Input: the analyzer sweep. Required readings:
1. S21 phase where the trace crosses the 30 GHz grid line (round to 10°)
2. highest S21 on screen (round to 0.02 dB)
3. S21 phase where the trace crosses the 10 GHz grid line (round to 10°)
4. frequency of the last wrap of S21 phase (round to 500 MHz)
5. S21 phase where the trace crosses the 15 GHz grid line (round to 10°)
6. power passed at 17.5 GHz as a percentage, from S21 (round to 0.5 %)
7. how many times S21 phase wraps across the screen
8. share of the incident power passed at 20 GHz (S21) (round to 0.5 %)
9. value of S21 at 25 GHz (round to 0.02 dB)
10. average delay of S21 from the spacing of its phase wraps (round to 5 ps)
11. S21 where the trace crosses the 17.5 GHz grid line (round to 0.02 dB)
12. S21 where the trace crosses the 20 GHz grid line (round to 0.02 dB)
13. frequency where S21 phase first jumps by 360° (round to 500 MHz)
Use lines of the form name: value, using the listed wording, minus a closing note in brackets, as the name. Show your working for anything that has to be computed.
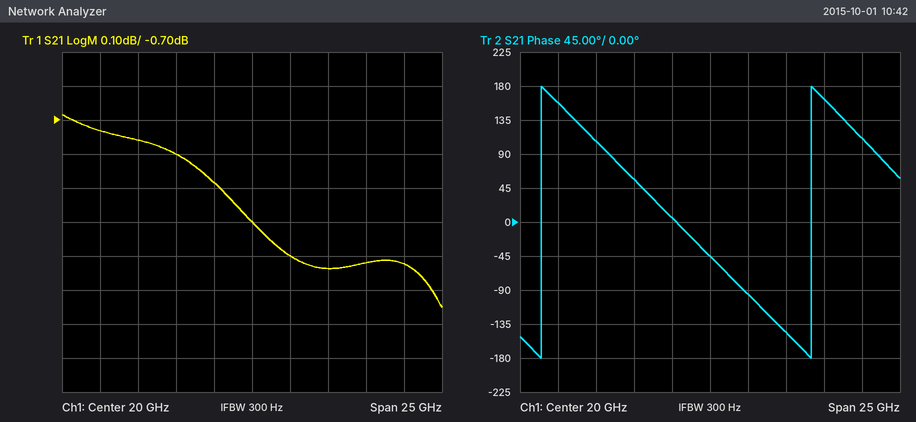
S21 phase where the trace crosses the 30 GHz grid line: 110°
highest S21 on screen: -0.68 dB
S21 phase where the trace crosses the 10 GHz grid line: 160°
frequency of the last wrap of S21 phase: 26.5 GHz
S21 phase where the trace crosses the 15 GHz grid line: 60°
power passed at 17.5 GHz as a percentage, from S21: 10^(-0.88/10) ≈ 81.7 %, so 81.5 % to the nearest 0.5 %
how many times S21 phase wraps across the screen: 2
share of the incident power passed at 20 GHz (S21): 10^(-1/10) ≈ 79.4 %, so 79.5 % to the nearest 0.5 %
value of S21 at 25 GHz: -1.14 dB
average delay of S21 from the spacing of its phase wraps: 1 cycle / (26.5 GHz − 9.0 GHz) ≈ 57.1 ps, so 55 ps to the nearest 5 ps
S21 where the trace crosses the 17.5 GHz grid line: -0.88 dB
S21 where the trace crosses the 20 GHz grid line: -1.00 dB
frequency where S21 phase first jumps by 360°: 9.0 GHz
